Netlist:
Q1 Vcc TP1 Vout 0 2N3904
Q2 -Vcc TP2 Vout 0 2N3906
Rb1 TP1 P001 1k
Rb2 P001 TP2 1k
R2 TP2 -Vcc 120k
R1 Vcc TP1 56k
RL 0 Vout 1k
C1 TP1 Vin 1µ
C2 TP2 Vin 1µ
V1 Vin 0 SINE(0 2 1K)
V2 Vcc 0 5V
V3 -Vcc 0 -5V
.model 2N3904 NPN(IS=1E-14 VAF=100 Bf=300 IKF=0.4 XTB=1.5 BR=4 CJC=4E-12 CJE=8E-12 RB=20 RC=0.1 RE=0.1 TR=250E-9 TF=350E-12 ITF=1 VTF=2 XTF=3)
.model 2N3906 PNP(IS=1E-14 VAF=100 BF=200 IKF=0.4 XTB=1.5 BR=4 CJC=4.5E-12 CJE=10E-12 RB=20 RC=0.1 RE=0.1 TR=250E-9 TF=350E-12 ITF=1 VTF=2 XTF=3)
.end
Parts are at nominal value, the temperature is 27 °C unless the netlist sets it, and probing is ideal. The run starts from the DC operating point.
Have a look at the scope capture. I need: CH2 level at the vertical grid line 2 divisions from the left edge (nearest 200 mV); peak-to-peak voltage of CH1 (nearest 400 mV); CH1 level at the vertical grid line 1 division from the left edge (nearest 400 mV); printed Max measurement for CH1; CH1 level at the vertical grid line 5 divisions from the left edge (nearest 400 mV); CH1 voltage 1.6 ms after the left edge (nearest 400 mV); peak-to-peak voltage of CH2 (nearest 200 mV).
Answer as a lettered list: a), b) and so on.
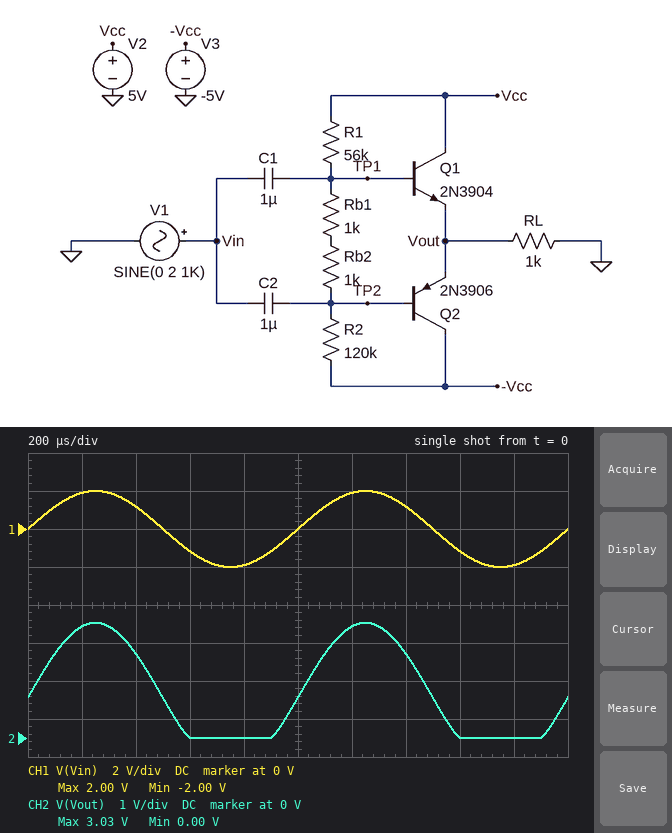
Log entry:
a) 2.2 V
b) 4.0 V
c) 2.0 V
d) 2.00 V
e) 0 V
f) -1.2 V
g) 3.0 V
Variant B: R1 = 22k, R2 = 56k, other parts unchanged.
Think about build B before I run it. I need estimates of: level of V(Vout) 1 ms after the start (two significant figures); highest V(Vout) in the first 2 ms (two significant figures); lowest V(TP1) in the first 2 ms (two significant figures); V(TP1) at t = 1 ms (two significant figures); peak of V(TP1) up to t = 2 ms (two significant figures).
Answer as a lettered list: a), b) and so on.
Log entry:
a) 1.5 V
b) 3.5 V
c) 160 mV
d) 2.2 V
e) 4.2 V
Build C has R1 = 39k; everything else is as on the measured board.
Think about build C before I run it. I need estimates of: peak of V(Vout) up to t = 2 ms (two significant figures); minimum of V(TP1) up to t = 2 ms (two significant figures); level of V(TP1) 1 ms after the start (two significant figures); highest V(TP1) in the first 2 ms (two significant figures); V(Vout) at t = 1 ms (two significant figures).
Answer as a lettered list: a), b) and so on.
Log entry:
a) 3.7 V
b) 400 mV
c) 2.4 V
d) 4.4 V
e) 1.7 V
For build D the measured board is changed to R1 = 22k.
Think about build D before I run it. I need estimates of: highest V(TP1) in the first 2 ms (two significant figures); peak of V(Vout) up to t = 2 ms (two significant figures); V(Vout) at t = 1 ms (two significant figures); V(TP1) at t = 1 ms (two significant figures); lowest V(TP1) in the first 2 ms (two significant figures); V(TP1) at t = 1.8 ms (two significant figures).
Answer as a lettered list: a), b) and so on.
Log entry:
a) 5.3 V
b) 4.6 V
c) 2.6 V
d) 3.3 V
e) 1.3 V
f) 1.4 V
